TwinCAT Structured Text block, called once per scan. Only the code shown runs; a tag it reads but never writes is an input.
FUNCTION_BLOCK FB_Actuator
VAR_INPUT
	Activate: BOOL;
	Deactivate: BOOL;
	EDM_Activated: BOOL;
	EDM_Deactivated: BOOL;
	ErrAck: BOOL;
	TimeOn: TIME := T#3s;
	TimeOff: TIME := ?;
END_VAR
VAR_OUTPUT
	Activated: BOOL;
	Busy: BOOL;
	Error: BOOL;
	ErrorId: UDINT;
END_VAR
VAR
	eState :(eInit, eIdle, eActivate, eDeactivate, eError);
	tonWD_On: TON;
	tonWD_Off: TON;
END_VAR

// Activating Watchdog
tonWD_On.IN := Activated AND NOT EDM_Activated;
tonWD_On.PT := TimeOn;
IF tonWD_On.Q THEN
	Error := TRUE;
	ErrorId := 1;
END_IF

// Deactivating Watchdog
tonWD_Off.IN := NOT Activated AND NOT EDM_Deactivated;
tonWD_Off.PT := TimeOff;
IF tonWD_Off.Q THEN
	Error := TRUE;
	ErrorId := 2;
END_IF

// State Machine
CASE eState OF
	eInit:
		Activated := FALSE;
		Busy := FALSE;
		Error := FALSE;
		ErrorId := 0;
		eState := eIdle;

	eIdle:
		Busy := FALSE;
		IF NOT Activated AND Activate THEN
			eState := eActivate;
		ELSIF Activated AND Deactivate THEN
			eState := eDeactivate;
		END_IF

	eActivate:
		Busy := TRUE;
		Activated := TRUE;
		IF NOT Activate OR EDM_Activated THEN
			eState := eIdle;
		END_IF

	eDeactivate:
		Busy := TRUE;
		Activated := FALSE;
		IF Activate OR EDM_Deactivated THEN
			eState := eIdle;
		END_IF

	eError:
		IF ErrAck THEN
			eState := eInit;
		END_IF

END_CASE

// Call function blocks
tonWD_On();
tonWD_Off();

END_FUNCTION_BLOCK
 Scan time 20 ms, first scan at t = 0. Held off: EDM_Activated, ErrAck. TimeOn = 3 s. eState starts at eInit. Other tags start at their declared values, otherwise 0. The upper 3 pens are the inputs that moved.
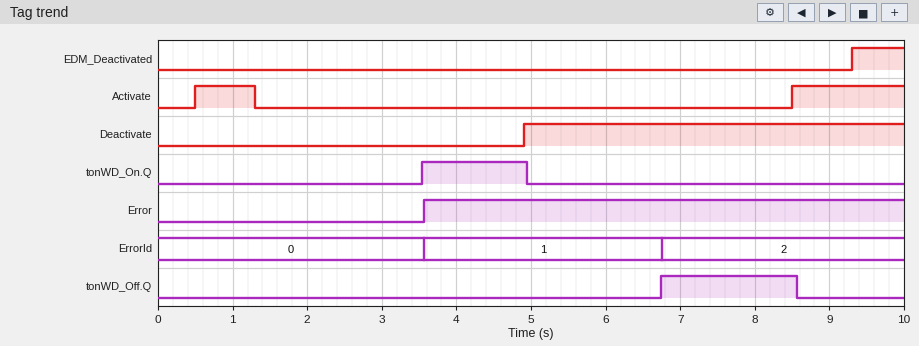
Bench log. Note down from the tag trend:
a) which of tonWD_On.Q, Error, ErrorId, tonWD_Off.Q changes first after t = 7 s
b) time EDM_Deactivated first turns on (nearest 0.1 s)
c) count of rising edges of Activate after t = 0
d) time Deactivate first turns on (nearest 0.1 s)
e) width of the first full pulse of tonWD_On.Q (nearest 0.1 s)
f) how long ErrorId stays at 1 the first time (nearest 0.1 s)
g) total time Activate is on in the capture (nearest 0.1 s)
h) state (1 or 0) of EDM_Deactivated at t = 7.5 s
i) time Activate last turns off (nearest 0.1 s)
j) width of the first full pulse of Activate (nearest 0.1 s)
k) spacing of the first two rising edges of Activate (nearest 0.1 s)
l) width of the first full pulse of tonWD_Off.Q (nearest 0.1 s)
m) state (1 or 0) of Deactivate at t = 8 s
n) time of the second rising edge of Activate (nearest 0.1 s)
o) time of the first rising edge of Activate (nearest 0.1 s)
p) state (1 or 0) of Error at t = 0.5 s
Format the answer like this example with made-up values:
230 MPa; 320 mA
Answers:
tonWD_Off.Q; 9.3 s; 2; 4.9 s; 1.4 s; 3.2 s; 2.3 s; 0; 1.3 s; 0.8 s; 8.0 s; 1.8 s; 1; 8.5 s; 0.5 s; 0
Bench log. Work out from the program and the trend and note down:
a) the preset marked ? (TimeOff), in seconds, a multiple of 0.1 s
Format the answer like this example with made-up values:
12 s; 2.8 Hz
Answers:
1.8 s
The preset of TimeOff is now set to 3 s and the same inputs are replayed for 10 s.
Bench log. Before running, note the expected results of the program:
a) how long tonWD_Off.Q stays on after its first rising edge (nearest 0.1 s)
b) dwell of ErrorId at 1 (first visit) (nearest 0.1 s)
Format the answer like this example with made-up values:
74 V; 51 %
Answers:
0.6 s; 4.4 s
